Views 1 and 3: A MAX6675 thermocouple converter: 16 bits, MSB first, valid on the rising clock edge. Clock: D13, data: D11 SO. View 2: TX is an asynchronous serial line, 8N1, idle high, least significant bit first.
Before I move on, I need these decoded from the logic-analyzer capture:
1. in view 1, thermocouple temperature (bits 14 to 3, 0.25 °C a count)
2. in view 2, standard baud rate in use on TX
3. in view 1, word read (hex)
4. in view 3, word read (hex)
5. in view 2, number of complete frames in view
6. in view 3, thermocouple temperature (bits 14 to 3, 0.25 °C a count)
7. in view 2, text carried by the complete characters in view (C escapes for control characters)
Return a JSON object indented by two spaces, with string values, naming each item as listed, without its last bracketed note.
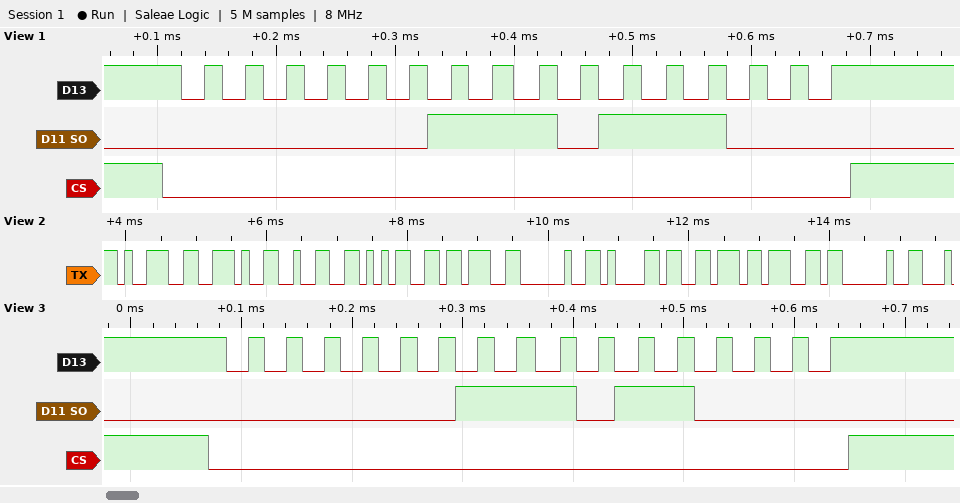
{
  "in view 1, thermocouple temperature": "29.75 °C",
  "in view 2, standard baud rate in use on TX": "9600 baud",
  "in view 1, word read": "0x03B8",
  "in view 3, word read": "0x03B0",
  "in view 2, number of complete frames in view": "10",
  "in view 3, thermocouple temperature": "29.50 °C",
  "in view 2, text carried by the complete characters in view": "\"9.25; avg \""
}
